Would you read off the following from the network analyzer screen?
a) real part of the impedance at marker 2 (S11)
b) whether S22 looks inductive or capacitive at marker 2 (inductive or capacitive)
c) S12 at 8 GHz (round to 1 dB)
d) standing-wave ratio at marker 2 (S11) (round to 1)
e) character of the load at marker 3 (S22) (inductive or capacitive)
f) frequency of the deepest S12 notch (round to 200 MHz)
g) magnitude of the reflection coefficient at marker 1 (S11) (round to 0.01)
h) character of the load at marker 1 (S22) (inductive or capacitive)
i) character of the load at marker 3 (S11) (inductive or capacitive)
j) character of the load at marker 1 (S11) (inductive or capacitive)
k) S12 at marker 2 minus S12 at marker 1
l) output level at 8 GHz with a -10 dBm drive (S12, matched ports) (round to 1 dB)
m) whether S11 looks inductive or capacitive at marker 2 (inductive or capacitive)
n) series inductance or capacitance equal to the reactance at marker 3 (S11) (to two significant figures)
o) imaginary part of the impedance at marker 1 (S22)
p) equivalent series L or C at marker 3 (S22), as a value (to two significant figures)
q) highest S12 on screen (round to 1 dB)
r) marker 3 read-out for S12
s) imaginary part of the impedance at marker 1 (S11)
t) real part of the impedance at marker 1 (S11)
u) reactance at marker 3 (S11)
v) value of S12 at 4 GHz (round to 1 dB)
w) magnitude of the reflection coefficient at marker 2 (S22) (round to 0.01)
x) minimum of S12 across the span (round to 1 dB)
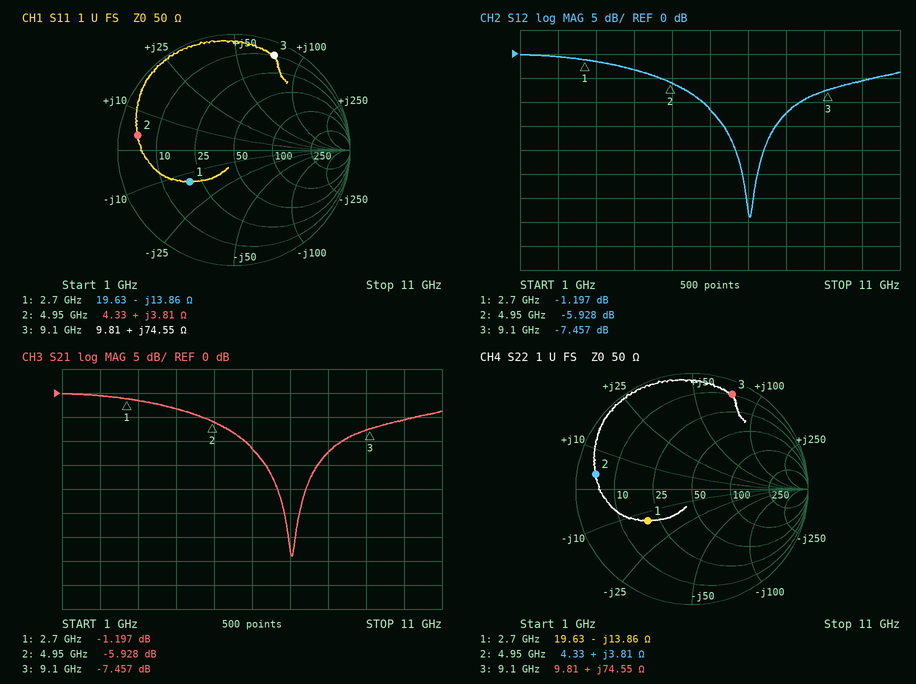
4.33 Ω
inductive
-12 dB
12
inductive
7.0 GHz
0.47
capacitive
inductive
capacitive
-4.731 dB
-22 dBm
inductive
1.3 nH
-13.86 Ω
1.3 nH
0 dB
-7.457 dB
-13.86 Ω
19.63 Ω
+74.55 Ω
-3 dB
0.84
-34 dB
